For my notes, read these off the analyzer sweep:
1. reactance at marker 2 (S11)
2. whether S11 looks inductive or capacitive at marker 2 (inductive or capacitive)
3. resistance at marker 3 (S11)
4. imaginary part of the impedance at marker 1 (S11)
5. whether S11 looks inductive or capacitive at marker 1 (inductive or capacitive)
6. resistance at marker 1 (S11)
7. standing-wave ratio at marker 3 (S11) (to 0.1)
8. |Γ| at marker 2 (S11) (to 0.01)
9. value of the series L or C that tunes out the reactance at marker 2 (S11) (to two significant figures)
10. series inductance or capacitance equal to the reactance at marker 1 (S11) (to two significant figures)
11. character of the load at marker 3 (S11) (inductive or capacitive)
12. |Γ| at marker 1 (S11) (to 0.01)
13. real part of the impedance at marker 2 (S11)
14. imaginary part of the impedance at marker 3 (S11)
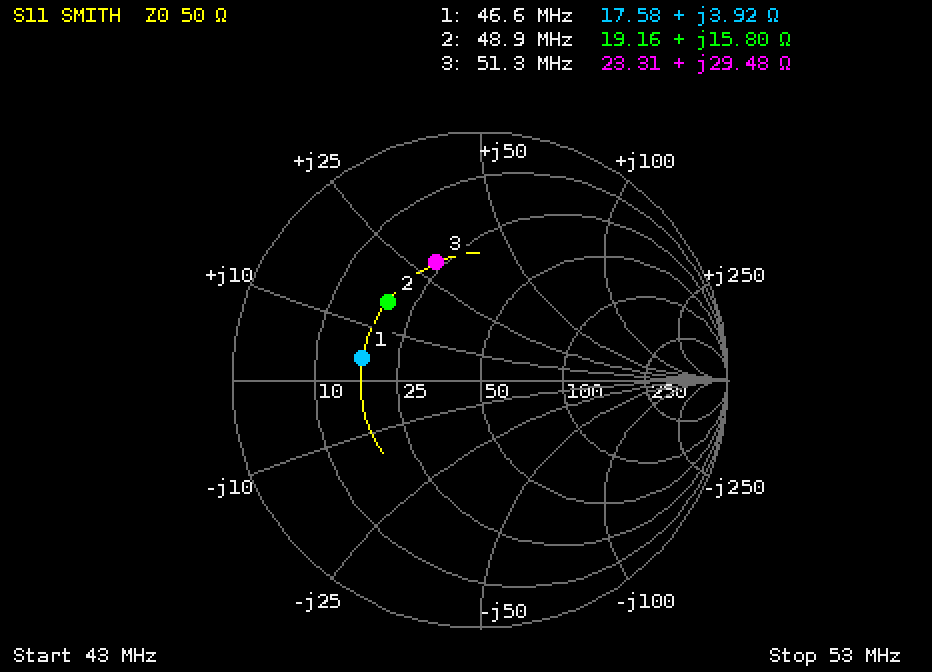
+15.80 Ω
inductive
23.31 Ω
+3.92 Ω
inductive
17.58 Ω
3.0
0.49
210 pF
13 nH
inductive
0.48
19.16 Ω
+29.48 Ω
